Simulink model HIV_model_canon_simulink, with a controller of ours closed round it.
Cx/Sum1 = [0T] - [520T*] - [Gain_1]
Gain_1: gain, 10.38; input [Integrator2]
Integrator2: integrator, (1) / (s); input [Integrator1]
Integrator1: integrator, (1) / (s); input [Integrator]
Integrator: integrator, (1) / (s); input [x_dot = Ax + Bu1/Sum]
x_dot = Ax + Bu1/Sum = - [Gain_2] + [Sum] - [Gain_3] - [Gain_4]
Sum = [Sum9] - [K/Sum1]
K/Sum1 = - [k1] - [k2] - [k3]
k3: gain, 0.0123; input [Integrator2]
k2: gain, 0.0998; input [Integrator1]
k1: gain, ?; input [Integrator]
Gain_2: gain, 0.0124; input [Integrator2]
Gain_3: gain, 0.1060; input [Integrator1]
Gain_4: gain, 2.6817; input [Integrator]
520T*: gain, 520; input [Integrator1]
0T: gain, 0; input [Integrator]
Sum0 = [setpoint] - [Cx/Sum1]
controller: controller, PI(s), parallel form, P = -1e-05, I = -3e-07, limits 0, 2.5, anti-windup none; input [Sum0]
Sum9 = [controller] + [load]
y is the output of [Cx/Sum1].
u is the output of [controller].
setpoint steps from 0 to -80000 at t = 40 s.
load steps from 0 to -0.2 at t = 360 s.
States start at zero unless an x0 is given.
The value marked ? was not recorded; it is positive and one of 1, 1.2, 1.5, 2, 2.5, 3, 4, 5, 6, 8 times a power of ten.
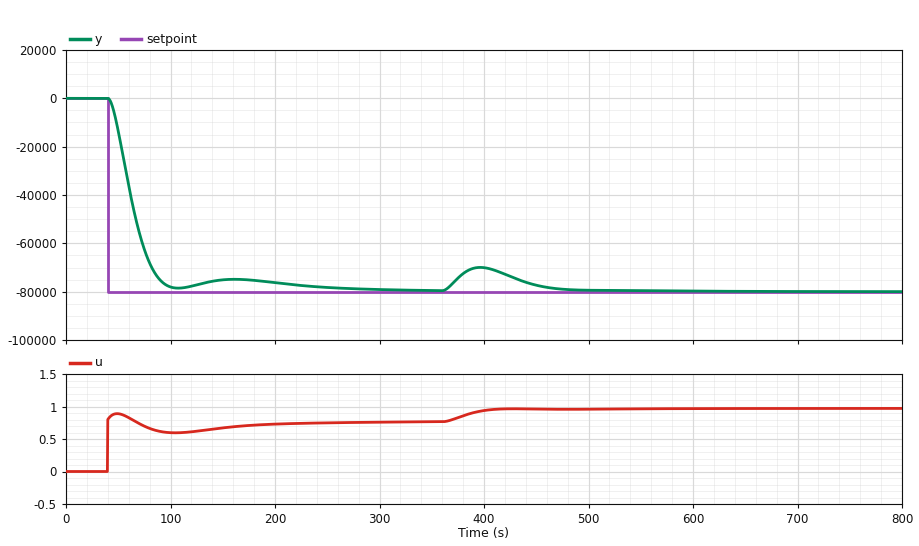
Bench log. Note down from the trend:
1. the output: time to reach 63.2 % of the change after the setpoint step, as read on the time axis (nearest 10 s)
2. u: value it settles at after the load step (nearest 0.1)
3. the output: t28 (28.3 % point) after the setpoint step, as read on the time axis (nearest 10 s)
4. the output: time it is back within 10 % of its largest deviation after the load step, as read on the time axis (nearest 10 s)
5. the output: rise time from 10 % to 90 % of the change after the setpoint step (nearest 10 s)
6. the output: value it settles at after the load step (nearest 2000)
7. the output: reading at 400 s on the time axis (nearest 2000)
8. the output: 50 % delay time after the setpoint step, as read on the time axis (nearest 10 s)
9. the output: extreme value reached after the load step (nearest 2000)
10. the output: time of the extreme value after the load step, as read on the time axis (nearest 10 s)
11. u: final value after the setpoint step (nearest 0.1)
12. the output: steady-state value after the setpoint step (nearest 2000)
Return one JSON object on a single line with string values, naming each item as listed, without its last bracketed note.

{"the output: time to reach 63.2 % of the change after the setpoint step, as read on the time axis": "70 s", "u: value it settles at after the load step": "1.0", "the output: t28 (28.3 % point) after the setpoint step, as read on the time axis": "50 s", "the output: time it is back within 10 % of its largest deviation after the load step, as read on the time axis": "480 s", "the output: rise time from 10 % to 90 % of the change after the setpoint step": "40 s", "the output: value it settles at after the load step": "-80000", "the output: reading at 400 s on the time axis": "-70000", "the output: 50 % delay time after the setpoint step, as read on the time axis": "60 s", "the output: extreme value reached after the load step": "-70000", "the output: time of the extreme value after the load step, as read on the time axis": "400 s", "u: final value after the setpoint step": "0.8", "the output: steady-state value after the setpoint step": "-80000"}
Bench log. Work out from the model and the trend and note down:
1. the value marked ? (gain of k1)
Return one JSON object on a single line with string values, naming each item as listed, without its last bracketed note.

{"the value marked ?": "2.5"}
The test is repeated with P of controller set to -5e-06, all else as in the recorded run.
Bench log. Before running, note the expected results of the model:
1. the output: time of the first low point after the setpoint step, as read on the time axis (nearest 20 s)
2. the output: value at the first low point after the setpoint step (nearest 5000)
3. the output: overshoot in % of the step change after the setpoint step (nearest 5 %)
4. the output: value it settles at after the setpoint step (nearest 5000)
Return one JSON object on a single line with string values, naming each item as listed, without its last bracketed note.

{"the output: time of the first low point after the setpoint step, as read on the time axis": "120 s", "the output: value at the first low point after the setpoint step": "-85000", "the output: overshoot in % of the step change after the setpoint step": "10 %", "the output: value it settles at after the setpoint step": "-80000"}
